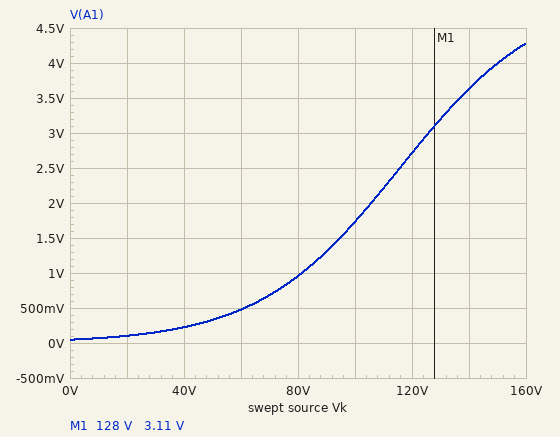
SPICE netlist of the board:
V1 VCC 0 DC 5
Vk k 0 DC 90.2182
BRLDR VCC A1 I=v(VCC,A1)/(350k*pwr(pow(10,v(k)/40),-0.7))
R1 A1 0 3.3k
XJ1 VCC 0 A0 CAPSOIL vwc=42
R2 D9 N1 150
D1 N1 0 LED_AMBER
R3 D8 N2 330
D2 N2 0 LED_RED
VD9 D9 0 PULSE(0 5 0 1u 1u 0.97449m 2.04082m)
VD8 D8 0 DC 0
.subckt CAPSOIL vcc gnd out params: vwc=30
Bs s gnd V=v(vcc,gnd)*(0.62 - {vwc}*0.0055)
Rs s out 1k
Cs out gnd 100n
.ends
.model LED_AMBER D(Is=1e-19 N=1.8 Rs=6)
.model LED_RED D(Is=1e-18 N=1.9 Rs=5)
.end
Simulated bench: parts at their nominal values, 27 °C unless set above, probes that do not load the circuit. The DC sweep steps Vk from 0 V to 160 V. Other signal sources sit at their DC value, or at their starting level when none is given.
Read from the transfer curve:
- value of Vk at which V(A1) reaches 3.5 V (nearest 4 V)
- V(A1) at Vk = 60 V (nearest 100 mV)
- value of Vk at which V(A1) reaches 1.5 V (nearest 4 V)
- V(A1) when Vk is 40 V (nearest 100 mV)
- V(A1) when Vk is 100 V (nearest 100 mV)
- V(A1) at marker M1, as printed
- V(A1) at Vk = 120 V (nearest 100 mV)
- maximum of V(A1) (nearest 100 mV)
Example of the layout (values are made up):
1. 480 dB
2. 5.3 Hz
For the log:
1. 136 V
2. 500 mV
3. 96 V
4. 200 mV
5. 1.7 V
6. 3.11 V
7. 2.7 V
8. 4.3 V
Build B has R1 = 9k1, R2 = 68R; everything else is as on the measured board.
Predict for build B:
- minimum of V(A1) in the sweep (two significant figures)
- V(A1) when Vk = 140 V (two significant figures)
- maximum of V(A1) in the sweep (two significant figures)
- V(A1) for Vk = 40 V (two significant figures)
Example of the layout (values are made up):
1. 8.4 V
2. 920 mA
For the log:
1. 130 mV
2. 4.4 V
3. 4.7 V
4. 580 mV
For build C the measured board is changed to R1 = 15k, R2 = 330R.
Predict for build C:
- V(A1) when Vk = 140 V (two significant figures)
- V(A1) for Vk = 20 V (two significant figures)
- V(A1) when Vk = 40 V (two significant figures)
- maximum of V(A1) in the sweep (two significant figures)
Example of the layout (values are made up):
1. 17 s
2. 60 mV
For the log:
1. 4.6 V
2. 440 mV
3. 880 mV
4. 4.8 V
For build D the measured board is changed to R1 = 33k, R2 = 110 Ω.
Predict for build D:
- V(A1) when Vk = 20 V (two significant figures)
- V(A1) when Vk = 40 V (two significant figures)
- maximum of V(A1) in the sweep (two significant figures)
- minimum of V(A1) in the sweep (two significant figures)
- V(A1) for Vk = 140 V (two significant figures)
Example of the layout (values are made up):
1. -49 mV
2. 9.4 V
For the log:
1. 870 mV
2. 1.6 V
3. 4.9 V
4. 430 mV
5. 4.8 V
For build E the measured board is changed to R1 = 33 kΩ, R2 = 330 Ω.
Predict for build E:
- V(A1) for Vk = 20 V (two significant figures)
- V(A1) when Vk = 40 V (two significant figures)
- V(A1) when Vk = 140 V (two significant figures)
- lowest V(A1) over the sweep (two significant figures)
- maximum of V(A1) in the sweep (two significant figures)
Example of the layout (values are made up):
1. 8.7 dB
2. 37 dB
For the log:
1. 870 mV
2. 1.6 V
3. 4.8 V
4. 430 mV
5. 4.9 V
